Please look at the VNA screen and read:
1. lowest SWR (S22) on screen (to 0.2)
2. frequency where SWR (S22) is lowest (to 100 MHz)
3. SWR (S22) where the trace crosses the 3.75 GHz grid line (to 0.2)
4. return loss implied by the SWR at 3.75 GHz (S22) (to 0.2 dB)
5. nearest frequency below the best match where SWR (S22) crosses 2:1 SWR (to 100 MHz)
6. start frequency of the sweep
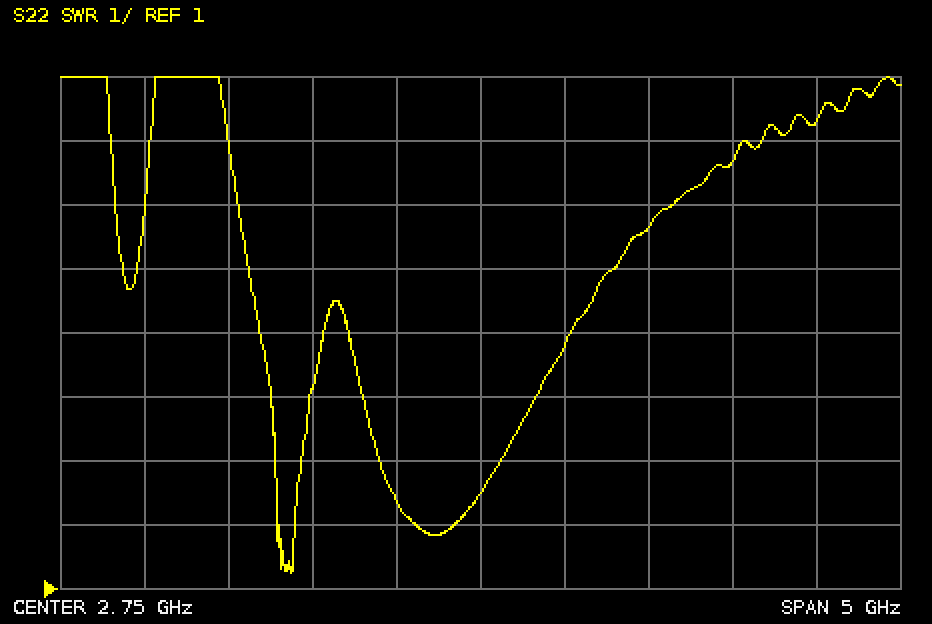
1.2
1.6 GHz
6.6
2.6 dB
1.5 GHz
250 MHz
